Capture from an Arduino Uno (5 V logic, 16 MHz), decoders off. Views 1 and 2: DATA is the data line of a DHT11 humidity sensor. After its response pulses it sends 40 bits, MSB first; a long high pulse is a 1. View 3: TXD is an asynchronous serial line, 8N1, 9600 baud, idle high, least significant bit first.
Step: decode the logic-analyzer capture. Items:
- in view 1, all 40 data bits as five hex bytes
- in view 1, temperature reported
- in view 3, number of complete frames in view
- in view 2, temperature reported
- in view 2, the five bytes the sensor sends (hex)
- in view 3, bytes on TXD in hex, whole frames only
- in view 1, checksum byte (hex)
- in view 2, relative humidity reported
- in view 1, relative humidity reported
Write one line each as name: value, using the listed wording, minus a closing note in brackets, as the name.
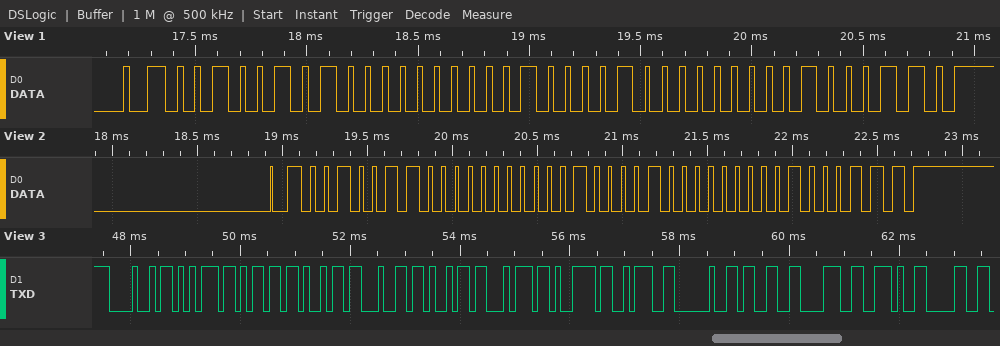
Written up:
in view 1, all 40 data bits as five hex bytes: 25 00 21 00 46
in view 1, temperature reported: 33.0 °C
in view 3, number of complete frames in view: 14
in view 2, temperature reported: 33.0 °C
in view 2, the five bytes the sensor sends: 26 00 21 00 47
in view 3, bytes on TXD in hex, whole frames only: 48 75 6D 69 64 69 74 79 3A 20 33 38 2E 30
in view 1, checksum byte: 0x46
in view 2, relative humidity reported: 38 %
in view 1, relative humidity reported: 37 %
